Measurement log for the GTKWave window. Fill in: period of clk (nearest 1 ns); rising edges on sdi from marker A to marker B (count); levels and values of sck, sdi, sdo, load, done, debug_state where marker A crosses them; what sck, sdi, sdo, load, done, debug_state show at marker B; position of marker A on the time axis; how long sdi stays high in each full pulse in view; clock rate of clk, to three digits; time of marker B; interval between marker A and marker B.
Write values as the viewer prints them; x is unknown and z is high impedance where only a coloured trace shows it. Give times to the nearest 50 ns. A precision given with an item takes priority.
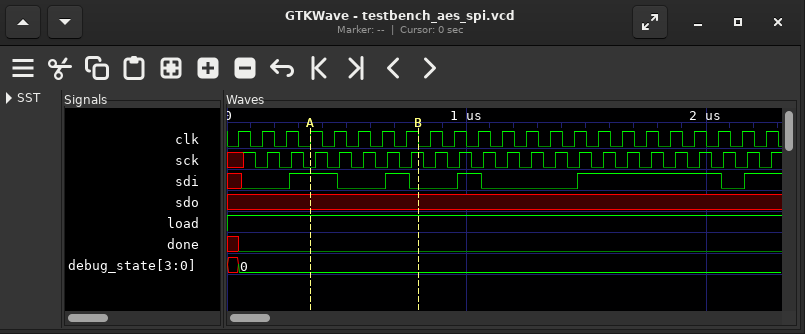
100 ns
1
sck=0, sdi=1, sdo=x, load=1, done=0, debug_state=0
sck=1, sdi=0, sdo=x, load=1, done=0, debug_state=0
350 ns
200 ns, 100 ns, 100 ns, 600 ns
10.0 MHz
800 ns
450 ns
